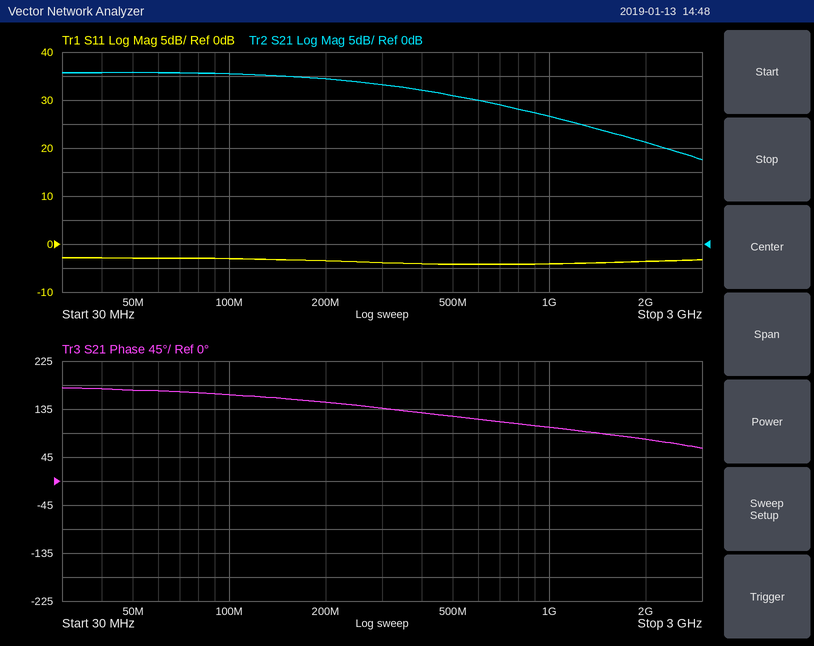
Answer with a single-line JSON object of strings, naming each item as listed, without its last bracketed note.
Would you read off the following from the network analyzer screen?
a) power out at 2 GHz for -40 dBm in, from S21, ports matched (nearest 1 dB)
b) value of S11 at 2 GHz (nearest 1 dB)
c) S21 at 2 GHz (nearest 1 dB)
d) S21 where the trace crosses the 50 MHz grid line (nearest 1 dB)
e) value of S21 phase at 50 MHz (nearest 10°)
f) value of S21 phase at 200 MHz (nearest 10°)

{"power out at 2 GHz for -40 dBm in, from S21, ports matched": "-19 dBm", "value of S11 at 2 GHz": "-4 dB", "S21 at 2 GHz": "21 dB", "S21 where the trace crosses the 50 MHz grid line": "36 dB", "value of S21 phase at 50 MHz": "170°", "value of S21 phase at 200 MHz": "150°"}
